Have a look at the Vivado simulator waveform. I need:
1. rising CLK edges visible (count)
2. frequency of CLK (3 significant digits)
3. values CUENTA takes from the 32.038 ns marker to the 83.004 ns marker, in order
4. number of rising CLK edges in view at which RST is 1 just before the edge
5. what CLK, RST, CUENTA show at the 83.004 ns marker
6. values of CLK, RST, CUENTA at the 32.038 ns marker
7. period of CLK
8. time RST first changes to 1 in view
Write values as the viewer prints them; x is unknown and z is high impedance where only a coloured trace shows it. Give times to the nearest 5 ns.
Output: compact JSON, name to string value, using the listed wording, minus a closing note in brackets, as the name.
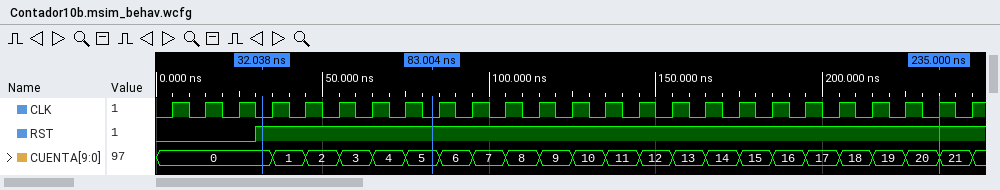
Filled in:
{"rising CLK edges visible": "25", "frequency of CLK": "100 MHz", "values CUENTA takes from the 32.038 ns marker to the 83.004 ns marker, in order": "0, 1, 2, 3, 4, 5", "number of rising CLK edges in view at which RST is 1 just before the edge": "22", "what CLK, RST, CUENTA show at the 83.004 ns marker": "CLK=0, RST=1, CUENTA=5", "values of CLK, RST, CUENTA at the 32.038 ns marker": "CLK=0, RST=1, CUENTA=0", "period of CLK": "10 ns", "time RST first changes to 1 in view": "30 ns"}
